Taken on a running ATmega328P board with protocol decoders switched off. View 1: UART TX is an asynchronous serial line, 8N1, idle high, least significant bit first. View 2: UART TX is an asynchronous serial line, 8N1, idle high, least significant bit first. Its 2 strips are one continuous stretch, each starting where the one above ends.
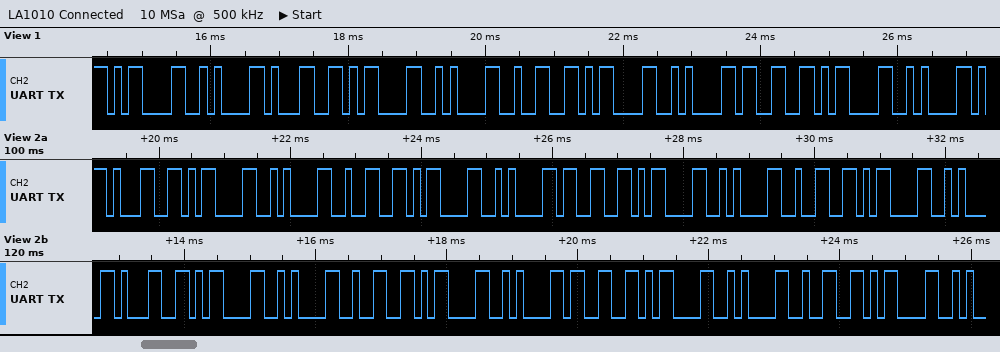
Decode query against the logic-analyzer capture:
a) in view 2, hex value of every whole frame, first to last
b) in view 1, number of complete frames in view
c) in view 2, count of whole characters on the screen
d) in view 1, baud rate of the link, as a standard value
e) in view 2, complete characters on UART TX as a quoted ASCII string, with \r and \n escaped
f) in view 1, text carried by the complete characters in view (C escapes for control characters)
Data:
31 0D 0A 32 0D 0A 33 0D 0A 32 0D 0A 31 0D 0A 32 0D 0A 33 0D 0A 32 0D
11
23
9600 baud
"1\r\n2\r\n3\r\n2\r\n1\r\n2\r\n3\r\n2\r"
"\r\n1\r\n2\r\n3\r\n"
